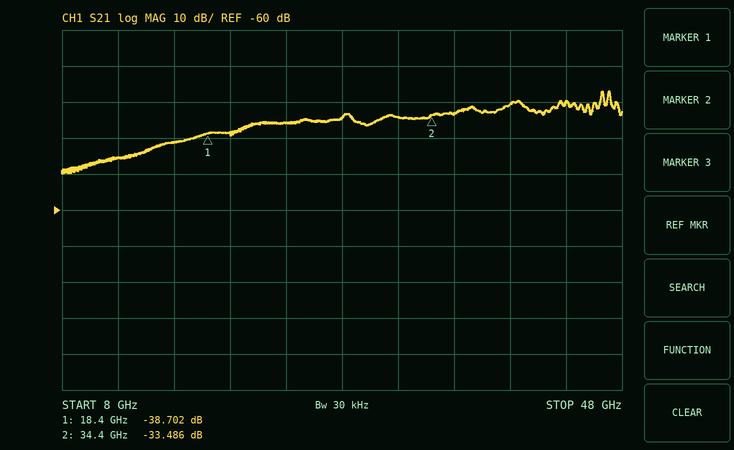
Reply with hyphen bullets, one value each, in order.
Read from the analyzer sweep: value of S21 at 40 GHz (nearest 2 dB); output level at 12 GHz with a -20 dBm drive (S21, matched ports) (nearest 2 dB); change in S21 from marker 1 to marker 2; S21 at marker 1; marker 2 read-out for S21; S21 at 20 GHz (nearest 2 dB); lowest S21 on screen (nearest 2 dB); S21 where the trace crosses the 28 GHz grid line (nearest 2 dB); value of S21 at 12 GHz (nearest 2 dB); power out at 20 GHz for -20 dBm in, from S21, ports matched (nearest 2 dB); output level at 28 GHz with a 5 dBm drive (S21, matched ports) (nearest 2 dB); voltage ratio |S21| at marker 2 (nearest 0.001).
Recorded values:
- -30 dB
- -66 dBm
- 5.216 dB
- -38.702 dB
- -33.486 dB
- -38 dB
- -50 dB
- -34 dB
- -46 dB
- -58 dBm
- -30 dBm
- 0.021
